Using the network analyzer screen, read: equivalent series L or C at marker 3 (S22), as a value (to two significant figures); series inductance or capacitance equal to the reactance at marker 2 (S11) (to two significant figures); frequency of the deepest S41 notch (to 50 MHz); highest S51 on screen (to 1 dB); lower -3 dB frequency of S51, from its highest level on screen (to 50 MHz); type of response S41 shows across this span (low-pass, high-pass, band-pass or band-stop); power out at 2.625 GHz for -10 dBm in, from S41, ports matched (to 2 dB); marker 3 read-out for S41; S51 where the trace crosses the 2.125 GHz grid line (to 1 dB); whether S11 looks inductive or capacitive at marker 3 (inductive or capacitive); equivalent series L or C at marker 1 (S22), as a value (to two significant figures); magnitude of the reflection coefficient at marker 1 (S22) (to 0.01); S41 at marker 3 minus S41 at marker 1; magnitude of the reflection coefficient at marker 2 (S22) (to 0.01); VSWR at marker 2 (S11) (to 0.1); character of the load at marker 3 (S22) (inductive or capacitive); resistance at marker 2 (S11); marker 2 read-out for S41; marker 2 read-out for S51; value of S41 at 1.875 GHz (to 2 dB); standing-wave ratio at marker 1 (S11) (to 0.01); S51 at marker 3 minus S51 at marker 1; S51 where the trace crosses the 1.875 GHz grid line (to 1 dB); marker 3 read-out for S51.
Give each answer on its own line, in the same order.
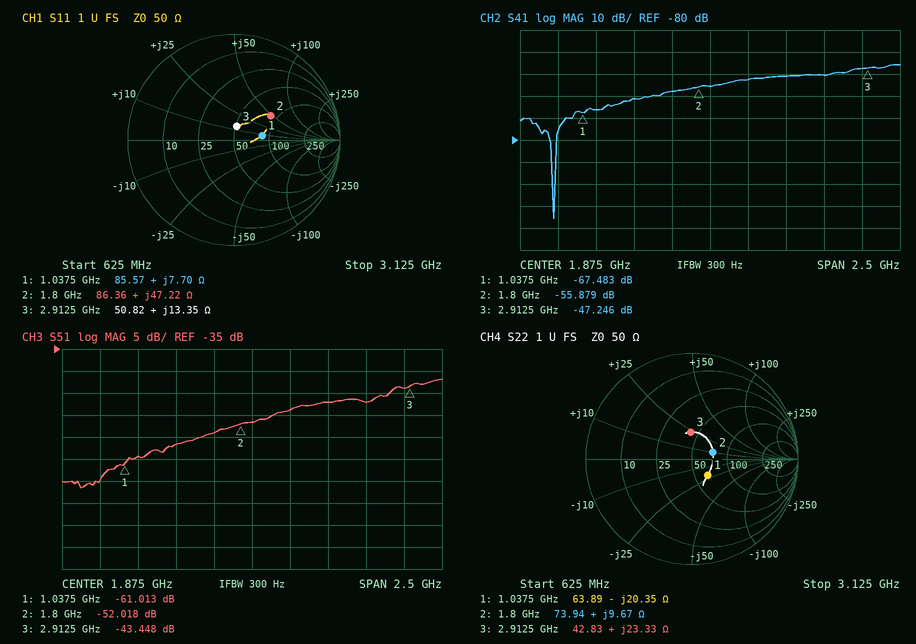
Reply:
1.3 nH
4.2 nH
850 MHz
-42 dB
2.80 GHz
high-pass
-60 dBm
-47.246 dB
-49 dB
inductive
7.5 pF
0.21
20.237 dB
0.21
2.4
inductive
86.36 Ω
-55.879 dB
-52.018 dB
-56 dB
1.73
17.565 dB
-52 dB
-43.448 dB
